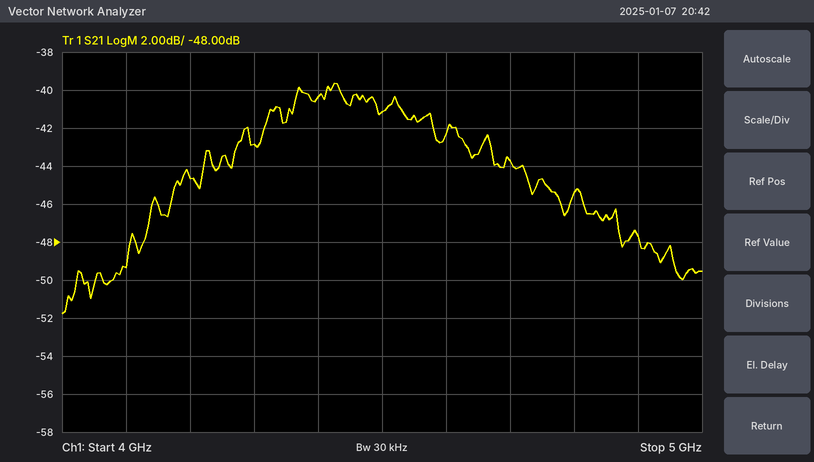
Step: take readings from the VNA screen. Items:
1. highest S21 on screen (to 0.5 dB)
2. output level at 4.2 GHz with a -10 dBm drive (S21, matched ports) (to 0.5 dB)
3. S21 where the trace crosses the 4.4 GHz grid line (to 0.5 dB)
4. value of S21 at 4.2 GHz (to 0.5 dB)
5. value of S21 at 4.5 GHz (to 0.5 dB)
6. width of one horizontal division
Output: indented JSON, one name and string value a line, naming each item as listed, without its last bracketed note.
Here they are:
{
  "highest S21 on screen": "-39.5 dB",
  "output level at 4.2 GHz with a -10 dBm drive (S21, matched ports)": "-54.5 dBm",
  "S21 where the trace crosses the 4.4 GHz grid line": "-40.5 dB",
  "value of S21 at 4.2 GHz": "-44.5 dB",
  "value of S21 at 4.5 GHz": "-41.0 dB",
  "width of one horizontal division": "100 MHz"
}
